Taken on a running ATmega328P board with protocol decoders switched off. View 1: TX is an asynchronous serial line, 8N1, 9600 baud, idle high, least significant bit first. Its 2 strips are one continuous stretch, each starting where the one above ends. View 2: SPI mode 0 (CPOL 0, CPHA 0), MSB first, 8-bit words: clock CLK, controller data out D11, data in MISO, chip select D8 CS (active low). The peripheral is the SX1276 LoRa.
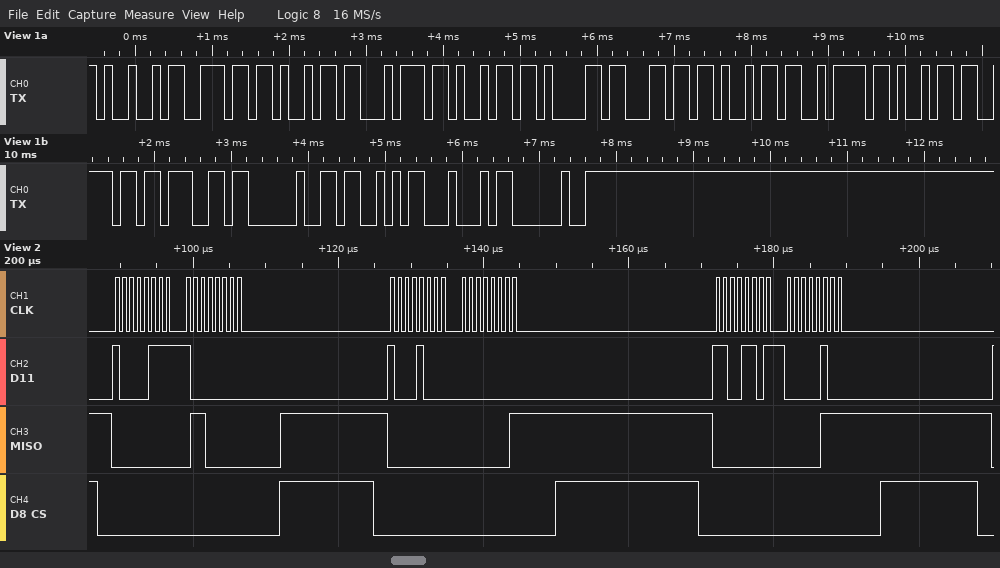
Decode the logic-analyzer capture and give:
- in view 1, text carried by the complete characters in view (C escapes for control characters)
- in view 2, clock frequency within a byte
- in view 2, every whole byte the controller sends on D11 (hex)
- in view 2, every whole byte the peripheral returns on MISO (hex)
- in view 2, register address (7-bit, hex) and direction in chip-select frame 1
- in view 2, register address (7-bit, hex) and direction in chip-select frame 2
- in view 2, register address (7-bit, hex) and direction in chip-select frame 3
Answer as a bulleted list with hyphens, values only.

- "Initializing SD "
- 1 MHz
- 87 80 88 00 CD 04
- 00 60 00 01 00 07
- 0x07 write
- 0x08 write
- 0x4D write
